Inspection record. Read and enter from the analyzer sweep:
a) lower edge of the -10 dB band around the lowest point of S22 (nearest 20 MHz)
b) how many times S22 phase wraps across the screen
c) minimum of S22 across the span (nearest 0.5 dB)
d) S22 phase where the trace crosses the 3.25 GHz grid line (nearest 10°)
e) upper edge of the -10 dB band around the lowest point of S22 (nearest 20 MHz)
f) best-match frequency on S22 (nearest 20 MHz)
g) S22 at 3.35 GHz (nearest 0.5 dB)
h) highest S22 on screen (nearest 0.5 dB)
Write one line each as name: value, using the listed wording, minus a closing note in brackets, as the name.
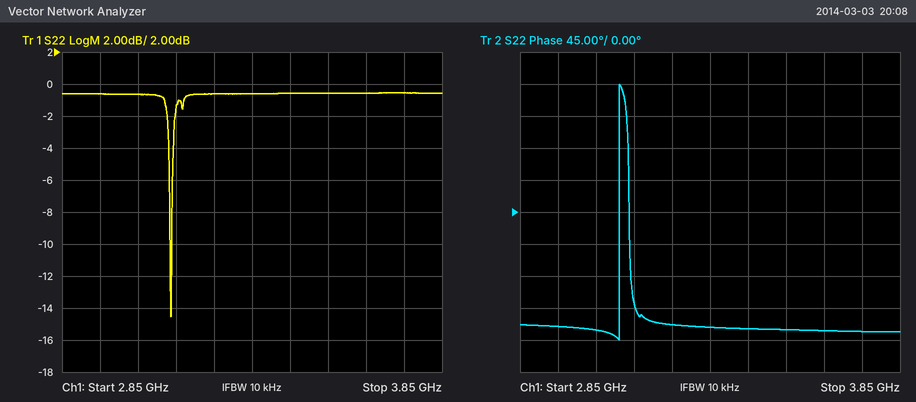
lower edge of the -10 dB band around the lowest point of S22: 3.14 GHz
how many times S22 phase wraps across the screen: 1
minimum of S22 across the span: -14.5 dB
S22 phase where the trace crosses the 3.25 GHz grid line: -160°
upper edge of the -10 dB band around the lowest point of S22: 3.14 GHz
best-match frequency on S22: 3.14 GHz
S22 at 3.35 GHz: -0.5 dB
highest S22 on screen: -0.5 dB
